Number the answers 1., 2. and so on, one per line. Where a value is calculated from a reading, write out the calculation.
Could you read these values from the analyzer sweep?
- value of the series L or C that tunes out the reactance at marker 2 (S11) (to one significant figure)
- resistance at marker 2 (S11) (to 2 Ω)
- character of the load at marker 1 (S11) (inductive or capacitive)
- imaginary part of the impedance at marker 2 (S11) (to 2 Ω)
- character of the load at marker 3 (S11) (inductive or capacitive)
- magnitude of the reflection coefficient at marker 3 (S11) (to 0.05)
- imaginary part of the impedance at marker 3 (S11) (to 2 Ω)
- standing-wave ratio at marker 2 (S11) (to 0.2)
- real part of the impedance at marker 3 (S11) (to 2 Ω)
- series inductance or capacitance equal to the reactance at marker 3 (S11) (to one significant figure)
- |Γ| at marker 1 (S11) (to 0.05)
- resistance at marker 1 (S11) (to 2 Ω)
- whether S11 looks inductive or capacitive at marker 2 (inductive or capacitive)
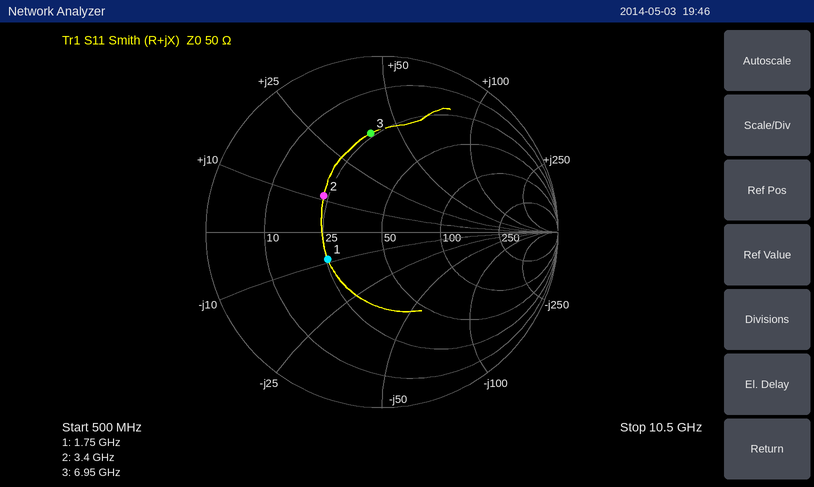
1. C = 1/(2π × 3.4 GHz × 12 Ω) ≈ 4 pF
2. 24 Ω
3. capacitive
4. +12 Ω
5. inductive
6. 0.55
7. +38 Ω
8. 2.2
9. 24 Ω
10. L = 38 Ω/(2π × 6.95 GHz) ≈ 870 pH, so 900 pH to one significant figure
11. 0.35
12. 26 Ω
13. inductive
